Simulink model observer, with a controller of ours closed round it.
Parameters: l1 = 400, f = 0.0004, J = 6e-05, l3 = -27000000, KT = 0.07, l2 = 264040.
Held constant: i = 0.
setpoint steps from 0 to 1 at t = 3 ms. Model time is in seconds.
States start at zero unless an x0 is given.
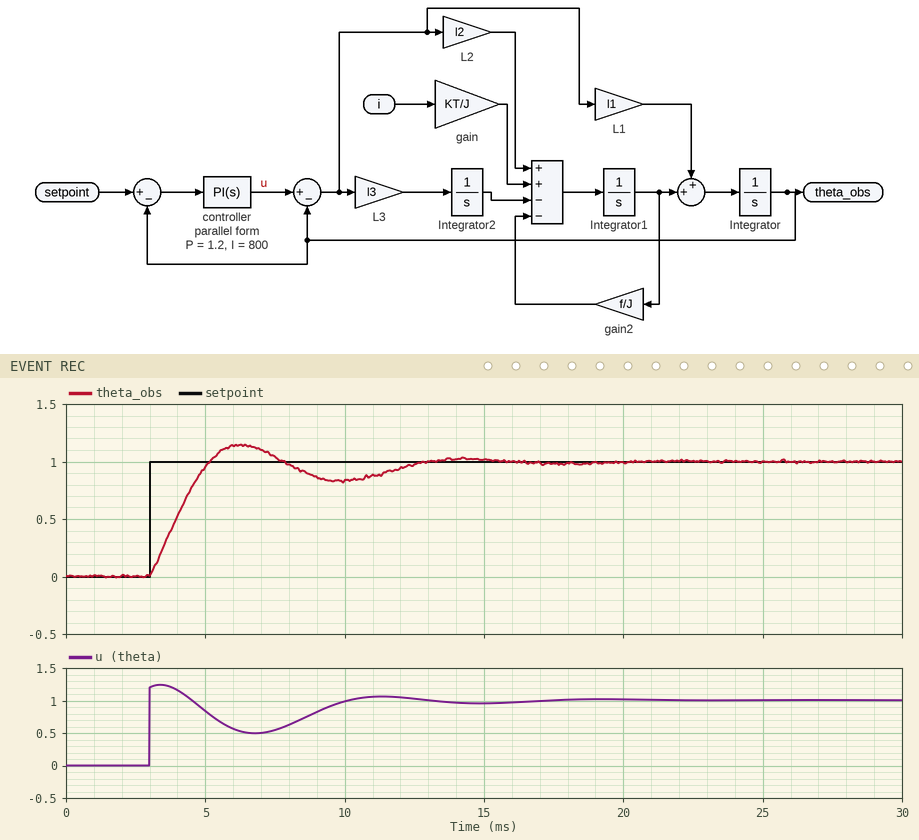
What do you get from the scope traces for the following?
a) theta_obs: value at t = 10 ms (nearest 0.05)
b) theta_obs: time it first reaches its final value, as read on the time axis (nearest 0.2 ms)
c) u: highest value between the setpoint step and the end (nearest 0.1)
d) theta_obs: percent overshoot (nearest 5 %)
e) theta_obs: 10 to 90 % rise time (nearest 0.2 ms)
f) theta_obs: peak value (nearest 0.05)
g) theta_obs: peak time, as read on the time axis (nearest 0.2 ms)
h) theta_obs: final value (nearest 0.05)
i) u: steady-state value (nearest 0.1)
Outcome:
0.85
5.2 ms
1.2
15 %
1.6 ms
1.15
6.2 ms
1.00
1.0
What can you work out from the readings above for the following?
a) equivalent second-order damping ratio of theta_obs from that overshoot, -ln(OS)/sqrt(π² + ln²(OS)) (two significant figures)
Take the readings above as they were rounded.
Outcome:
0.52
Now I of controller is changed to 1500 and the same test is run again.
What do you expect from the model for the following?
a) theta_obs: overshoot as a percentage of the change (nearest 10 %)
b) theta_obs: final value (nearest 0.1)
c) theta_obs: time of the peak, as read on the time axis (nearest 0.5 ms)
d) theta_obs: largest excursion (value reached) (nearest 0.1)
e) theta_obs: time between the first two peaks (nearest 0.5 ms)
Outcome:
30 %
1.0
6.0 ms
1.3
6.5 ms
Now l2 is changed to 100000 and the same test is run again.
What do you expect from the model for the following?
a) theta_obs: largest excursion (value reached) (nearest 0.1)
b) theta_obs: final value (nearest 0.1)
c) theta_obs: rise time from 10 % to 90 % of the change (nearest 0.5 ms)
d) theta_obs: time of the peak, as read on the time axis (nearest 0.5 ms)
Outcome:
1.2
1.0
2.0 ms
7.5 ms
